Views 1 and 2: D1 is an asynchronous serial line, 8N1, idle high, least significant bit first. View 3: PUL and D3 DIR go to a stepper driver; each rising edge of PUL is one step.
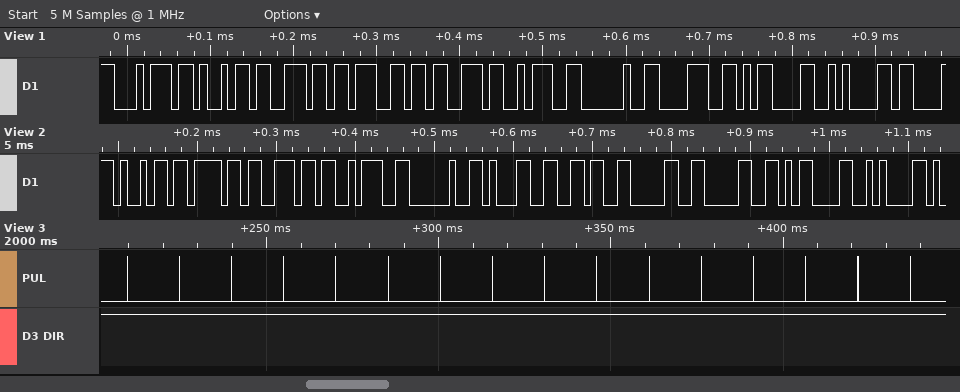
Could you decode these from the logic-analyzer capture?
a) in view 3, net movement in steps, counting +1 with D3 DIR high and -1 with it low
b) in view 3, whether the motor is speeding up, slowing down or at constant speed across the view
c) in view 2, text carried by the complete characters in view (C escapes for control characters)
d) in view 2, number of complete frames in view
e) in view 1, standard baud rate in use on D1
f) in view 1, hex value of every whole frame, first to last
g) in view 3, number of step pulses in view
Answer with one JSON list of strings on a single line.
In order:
["+16", "constant speed", "\"ion: 1600\\r\\n\"", "11", "115200 baud", "74 69 6E 67 73 3A 20 38 0D 0A", "16"]
